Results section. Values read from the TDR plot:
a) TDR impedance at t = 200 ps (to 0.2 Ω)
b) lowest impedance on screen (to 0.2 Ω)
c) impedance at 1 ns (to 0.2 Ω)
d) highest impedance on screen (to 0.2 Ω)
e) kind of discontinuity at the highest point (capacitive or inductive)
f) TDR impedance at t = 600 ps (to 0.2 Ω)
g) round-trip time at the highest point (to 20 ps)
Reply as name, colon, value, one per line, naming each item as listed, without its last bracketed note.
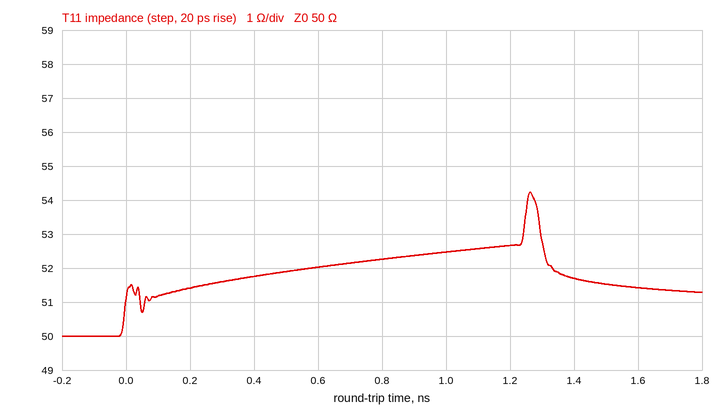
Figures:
TDR impedance at t = 200 ps: 51.4 Ω
lowest impedance on screen: 50.0 Ω
impedance at 1 ns: 52.4 Ω
highest impedance on screen: 54.2 Ω
kind of discontinuity at the highest point: inductive
TDR impedance at t = 600 ps: 52.0 Ω
round-trip time at the highest point: 1.26 ns
